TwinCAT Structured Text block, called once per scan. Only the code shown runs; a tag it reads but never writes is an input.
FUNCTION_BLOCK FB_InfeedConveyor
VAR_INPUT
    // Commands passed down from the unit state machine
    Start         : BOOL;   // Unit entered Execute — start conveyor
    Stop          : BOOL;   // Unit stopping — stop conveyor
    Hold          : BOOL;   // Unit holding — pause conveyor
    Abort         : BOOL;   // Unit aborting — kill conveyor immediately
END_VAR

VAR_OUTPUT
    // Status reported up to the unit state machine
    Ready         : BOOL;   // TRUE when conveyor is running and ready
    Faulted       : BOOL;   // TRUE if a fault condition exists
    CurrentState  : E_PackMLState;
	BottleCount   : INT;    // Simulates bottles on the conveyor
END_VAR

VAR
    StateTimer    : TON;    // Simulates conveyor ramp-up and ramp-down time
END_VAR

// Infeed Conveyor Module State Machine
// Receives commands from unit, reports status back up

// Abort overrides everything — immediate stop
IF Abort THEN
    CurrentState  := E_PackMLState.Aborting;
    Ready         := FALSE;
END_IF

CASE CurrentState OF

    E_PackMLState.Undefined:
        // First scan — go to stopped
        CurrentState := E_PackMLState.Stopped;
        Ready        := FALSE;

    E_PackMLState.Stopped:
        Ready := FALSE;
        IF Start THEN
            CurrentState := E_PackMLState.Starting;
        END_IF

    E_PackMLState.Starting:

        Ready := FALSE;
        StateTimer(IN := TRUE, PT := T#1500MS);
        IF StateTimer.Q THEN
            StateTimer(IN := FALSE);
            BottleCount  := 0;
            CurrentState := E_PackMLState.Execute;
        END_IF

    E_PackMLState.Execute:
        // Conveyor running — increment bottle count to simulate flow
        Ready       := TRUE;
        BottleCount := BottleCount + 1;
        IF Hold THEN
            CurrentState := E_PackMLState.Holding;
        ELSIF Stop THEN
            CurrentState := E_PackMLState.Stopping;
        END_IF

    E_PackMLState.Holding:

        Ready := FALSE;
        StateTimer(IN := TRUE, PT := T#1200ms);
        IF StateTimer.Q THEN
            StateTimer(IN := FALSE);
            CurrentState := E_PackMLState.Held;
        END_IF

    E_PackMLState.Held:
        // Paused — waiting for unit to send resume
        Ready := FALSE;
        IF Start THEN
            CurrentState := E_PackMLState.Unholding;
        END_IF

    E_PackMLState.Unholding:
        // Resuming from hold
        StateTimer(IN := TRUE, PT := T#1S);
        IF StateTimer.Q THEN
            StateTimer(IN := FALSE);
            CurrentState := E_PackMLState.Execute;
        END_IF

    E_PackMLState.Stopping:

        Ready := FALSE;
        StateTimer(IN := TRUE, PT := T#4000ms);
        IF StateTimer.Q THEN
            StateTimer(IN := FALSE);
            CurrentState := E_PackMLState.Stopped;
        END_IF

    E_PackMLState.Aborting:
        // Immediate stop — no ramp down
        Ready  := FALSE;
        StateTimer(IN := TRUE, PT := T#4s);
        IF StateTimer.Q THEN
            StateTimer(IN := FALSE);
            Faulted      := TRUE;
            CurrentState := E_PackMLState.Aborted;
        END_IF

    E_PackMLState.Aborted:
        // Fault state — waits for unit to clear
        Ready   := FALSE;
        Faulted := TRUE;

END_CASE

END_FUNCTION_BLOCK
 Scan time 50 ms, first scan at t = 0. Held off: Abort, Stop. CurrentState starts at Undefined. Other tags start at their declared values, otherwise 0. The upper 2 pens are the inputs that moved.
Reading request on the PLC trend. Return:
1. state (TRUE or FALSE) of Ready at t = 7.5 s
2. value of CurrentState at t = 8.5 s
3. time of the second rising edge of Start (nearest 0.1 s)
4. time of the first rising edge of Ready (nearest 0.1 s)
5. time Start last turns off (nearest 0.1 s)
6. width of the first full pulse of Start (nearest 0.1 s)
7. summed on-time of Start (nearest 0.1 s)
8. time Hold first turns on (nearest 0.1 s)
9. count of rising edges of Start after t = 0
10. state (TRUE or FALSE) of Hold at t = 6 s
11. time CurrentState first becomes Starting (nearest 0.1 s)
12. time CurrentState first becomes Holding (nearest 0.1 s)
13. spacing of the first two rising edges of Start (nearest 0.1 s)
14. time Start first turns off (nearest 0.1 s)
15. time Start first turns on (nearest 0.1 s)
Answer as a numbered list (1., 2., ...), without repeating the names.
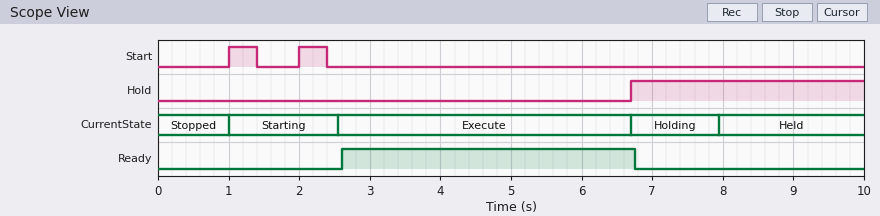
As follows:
1. FALSE
2. Held
3. 2.0 s
4. 2.6 s
5. 2.4 s
6. 0.4 s
7. 0.8 s
8. 6.7 s
9. 2
10. FALSE
11. 1.0 s
12. 6.7 s
13. 1.0 s
14. 1.4 s
15. 1.0 s
